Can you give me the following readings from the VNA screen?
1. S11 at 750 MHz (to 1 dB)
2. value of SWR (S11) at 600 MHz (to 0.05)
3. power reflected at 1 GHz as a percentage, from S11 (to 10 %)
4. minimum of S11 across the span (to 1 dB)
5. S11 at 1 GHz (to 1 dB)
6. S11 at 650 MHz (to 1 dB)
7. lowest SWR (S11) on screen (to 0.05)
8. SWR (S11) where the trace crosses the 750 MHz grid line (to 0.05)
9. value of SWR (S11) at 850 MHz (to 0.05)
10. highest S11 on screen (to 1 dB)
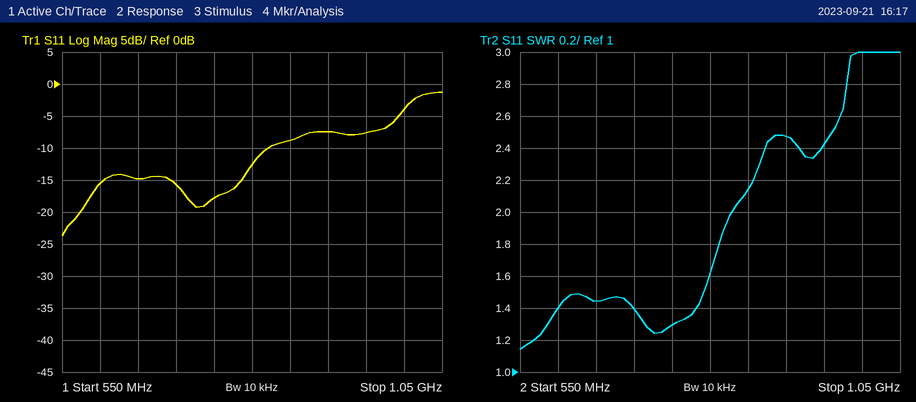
-18 dB
1.40
40 %
-24 dB
-4 dB
-15 dB
1.15
1.30
2.15
-1 dB
